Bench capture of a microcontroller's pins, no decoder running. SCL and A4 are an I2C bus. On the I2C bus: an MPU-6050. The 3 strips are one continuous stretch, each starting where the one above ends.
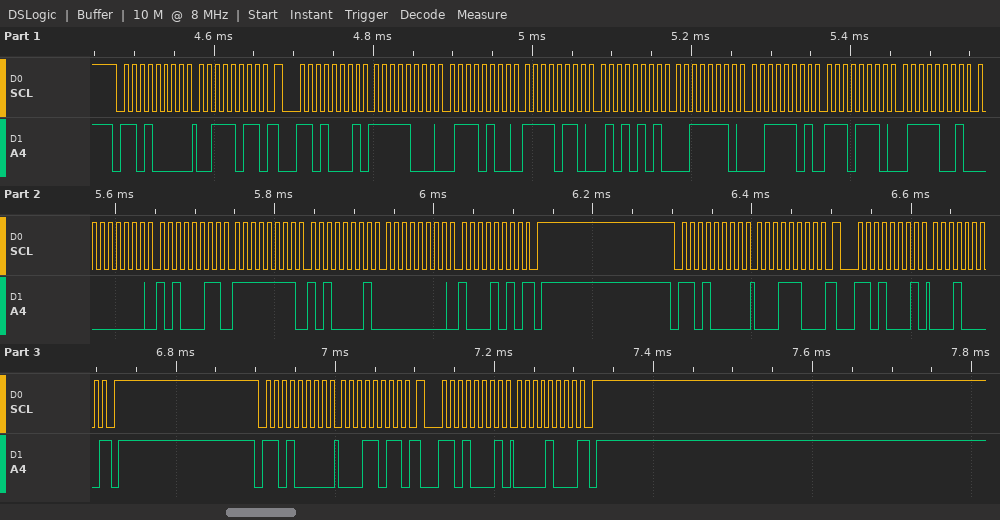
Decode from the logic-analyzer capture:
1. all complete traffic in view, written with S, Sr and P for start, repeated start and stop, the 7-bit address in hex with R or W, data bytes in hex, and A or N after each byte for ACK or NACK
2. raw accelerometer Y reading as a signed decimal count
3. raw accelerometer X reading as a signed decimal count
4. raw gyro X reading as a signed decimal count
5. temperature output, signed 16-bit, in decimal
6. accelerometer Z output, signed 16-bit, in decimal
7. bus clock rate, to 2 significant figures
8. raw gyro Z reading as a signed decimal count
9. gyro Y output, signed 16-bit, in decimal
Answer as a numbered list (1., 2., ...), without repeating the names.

1. S 68W A 3B A Sr 68R A F8 A 74 A F6 A 55 A 3E A 3D A EE A 79 A 00 A A3 A FF A A1 A 00 A 8A N P S 68W A 1C A Sr 68R A 10 N P S 68W A 1B A Sr 68R A 08 N P
2. -2475
3. -1932
4. 163
5. -4487
6. 15933
7. 100 kHz
8. 138
9. -95
